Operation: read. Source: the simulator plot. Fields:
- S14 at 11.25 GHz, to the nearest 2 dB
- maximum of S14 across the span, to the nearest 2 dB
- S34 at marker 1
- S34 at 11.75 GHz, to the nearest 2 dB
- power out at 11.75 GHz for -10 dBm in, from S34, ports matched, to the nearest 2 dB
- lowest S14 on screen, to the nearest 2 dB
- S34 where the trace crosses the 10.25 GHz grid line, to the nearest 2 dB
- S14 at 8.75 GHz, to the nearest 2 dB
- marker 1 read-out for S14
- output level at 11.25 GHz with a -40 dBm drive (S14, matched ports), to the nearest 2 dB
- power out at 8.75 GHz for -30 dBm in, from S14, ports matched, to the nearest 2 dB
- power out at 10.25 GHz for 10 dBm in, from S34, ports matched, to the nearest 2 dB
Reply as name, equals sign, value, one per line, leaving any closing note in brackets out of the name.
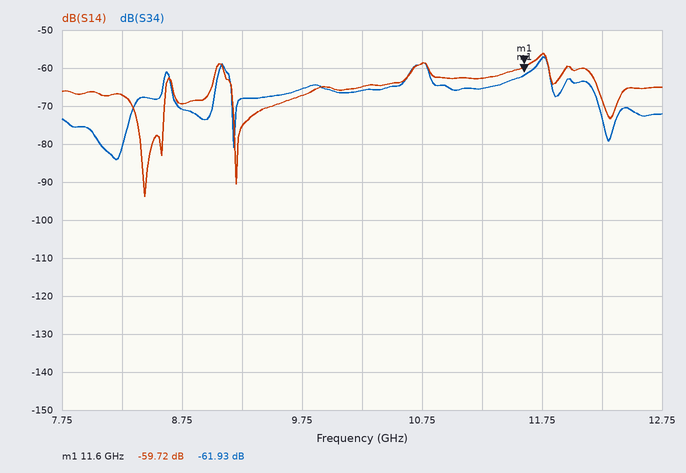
S14 at 11.25 GHz, to the nearest 2 dB = -62 dB
maximum of S14 across the span, to the nearest 2 dB = -56 dB
S34 at marker 1 = -61.93 dB
S34 at 11.75 GHz, to the nearest 2 dB = -58 dB
power out at 11.75 GHz for -10 dBm in, from S34, ports matched, to the nearest 2 dB = -68 dBm
lowest S14 on screen, to the nearest 2 dB = -94 dB
S34 where the trace crosses the 10.25 GHz grid line, to the nearest 2 dB = -66 dB
S14 at 8.75 GHz, to the nearest 2 dB = -70 dB
marker 1 read-out for S14 = -59.72 dB
output level at 11.25 GHz with a -40 dBm drive (S14, matched ports), to the nearest 2 dB = -102 dBm
power out at 8.75 GHz for -30 dBm in, from S14, ports matched, to the nearest 2 dB = -100 dBm
power out at 10.25 GHz for 10 dBm in, from S34, ports matched, to the nearest 2 dB = -56 dBm
